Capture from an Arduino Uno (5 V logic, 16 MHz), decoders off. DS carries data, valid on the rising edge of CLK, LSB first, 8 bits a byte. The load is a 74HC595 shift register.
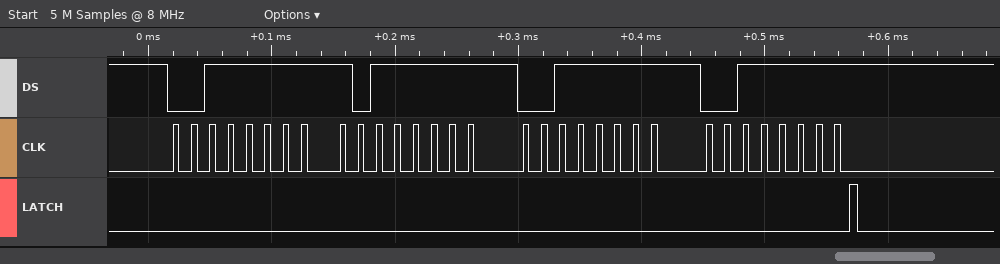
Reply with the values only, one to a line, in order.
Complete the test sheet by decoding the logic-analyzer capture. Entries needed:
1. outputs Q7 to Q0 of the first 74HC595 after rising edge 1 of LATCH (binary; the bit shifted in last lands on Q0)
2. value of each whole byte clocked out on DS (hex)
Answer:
00111111
0xFC 0xFD 0xFC 0xFC
